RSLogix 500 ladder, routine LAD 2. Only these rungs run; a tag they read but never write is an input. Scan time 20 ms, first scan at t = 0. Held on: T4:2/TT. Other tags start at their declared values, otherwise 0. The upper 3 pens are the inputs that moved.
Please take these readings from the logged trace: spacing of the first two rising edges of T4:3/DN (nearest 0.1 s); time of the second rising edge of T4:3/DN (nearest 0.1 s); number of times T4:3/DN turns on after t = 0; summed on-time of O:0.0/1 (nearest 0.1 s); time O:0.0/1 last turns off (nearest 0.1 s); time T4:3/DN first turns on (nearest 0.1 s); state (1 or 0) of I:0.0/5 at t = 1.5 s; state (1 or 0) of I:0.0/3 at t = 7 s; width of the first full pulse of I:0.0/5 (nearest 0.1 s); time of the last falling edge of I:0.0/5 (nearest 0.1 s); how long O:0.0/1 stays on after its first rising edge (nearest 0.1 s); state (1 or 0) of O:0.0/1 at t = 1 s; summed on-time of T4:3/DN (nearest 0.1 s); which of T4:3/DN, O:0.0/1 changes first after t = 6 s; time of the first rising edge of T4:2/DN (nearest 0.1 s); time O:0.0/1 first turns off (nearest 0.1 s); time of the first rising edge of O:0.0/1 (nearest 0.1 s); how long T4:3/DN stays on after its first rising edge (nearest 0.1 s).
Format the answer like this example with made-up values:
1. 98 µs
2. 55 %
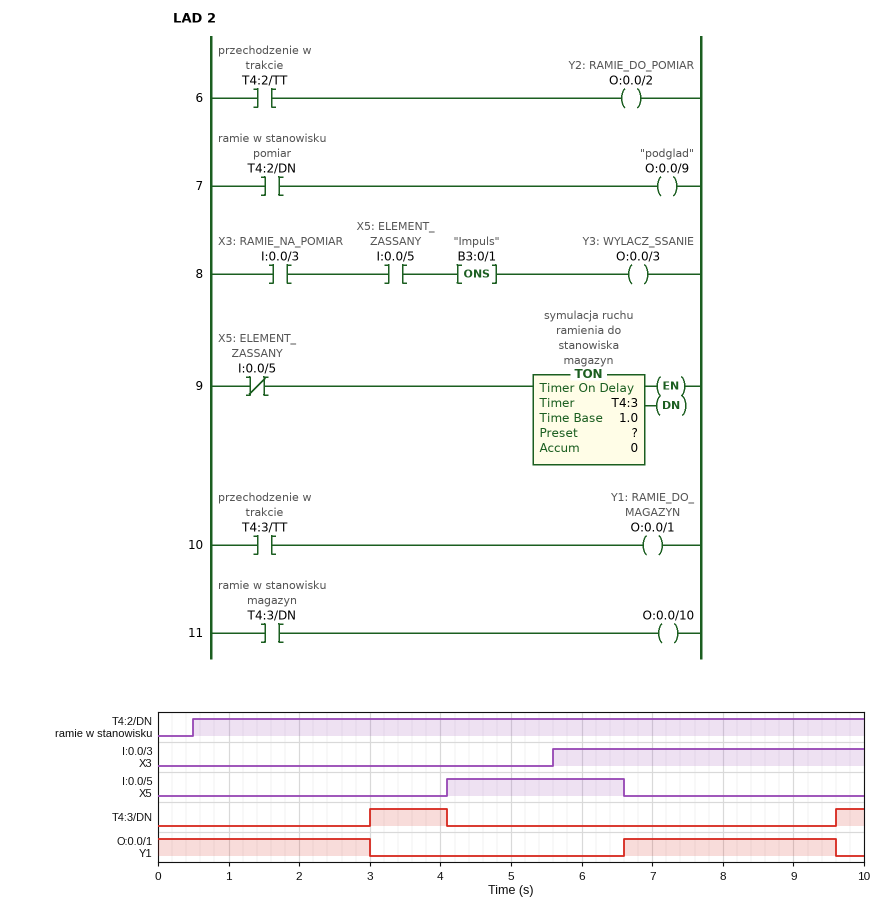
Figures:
1. 6.6 s
2. 9.6 s
3. 2
4. 6.0 s
5. 9.6 s
6. 3.0 s
7. 0
8. 1
9. 2.5 s
10. 6.6 s
11. 3.0 s
12. 1
13. 1.5 s
14. O:0.0/1
15. 0.5 s
16. 3.0 s
17. 6.6 s
18. 1.1 s
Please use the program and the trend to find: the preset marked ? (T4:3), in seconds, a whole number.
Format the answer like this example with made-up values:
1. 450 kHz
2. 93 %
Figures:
1. 3 s
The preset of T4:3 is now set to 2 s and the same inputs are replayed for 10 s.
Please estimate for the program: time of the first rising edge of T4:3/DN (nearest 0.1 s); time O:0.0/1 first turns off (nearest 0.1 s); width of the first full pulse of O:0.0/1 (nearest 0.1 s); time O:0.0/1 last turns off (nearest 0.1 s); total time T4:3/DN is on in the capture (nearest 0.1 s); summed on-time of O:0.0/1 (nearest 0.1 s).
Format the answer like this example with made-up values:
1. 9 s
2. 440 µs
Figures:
1. 2.0 s
2. 2.0 s
3. 2.0 s
4. 8.6 s
5. 3.5 s
6. 4.0 s
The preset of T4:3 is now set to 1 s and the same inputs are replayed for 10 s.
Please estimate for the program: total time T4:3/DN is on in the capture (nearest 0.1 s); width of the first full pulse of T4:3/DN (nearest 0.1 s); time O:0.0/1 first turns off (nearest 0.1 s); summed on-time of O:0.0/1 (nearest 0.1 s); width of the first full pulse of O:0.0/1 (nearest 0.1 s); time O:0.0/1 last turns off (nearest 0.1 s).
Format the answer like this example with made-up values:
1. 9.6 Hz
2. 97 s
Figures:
1. 5.5 s
2. 3.1 s
3. 1.0 s
4. 2.0 s
5. 1.0 s
6. 7.6 s
